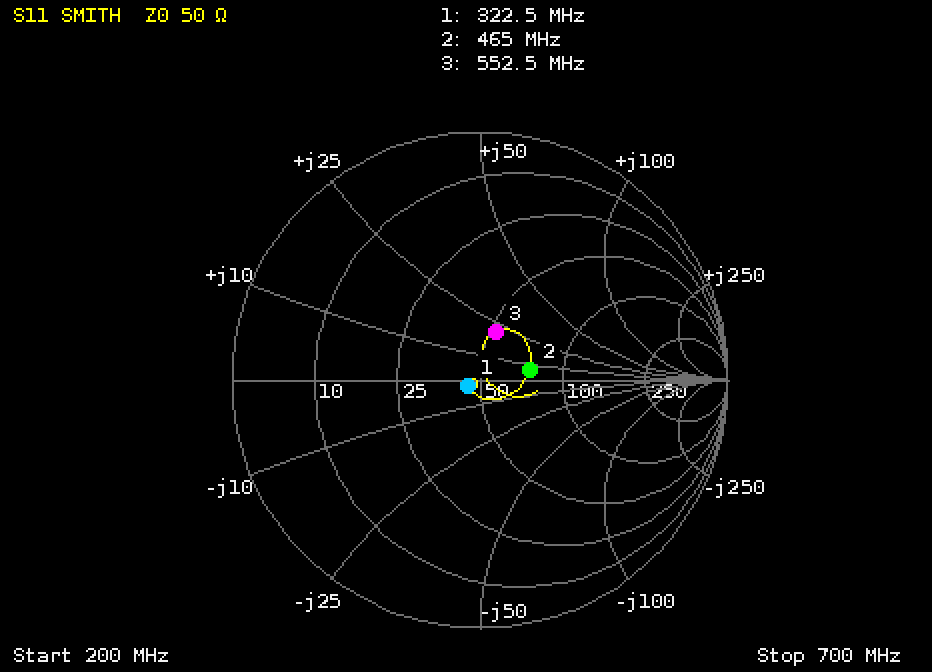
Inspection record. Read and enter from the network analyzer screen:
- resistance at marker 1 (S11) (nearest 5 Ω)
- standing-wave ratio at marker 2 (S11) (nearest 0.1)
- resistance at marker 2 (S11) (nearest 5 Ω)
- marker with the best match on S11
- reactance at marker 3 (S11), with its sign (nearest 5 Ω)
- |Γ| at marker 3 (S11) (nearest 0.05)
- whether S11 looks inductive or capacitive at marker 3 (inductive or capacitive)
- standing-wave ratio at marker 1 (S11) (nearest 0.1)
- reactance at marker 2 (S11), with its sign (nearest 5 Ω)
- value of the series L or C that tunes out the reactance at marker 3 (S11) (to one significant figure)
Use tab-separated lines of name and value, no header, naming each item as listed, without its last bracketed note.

resistance at marker 1 (S11)	45 Ω
standing-wave ratio at marker 2 (S11)	1.5
resistance at marker 2 (S11)	75 Ω
marker with the best match on S11	marker 1
reactance at marker 3 (S11), with its sign	+20 Ω
|Γ| at marker 3 (S11)	0.20
whether S11 looks inductive or capacitive at marker 3	inductive
standing-wave ratio at marker 1 (S11)	1.1
reactance at marker 2 (S11), with its sign	+5 Ω
value of the series L or C that tunes out the reactance at marker 3 (S11)	10 pF
